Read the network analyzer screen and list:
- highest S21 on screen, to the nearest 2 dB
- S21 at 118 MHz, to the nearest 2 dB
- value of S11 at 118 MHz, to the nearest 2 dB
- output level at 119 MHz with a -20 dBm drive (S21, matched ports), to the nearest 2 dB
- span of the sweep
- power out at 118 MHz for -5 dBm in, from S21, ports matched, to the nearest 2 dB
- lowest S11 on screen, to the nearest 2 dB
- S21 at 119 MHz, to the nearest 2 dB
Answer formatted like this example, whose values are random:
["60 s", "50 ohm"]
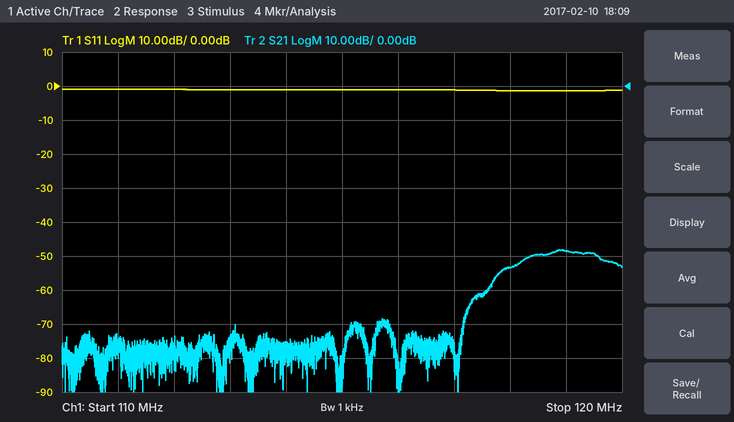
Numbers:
["-48 dB", "-54 dB", "-2 dB", "-68 dBm", "10 MHz", "-58 dBm", "-2 dB", "-48 dB"]
